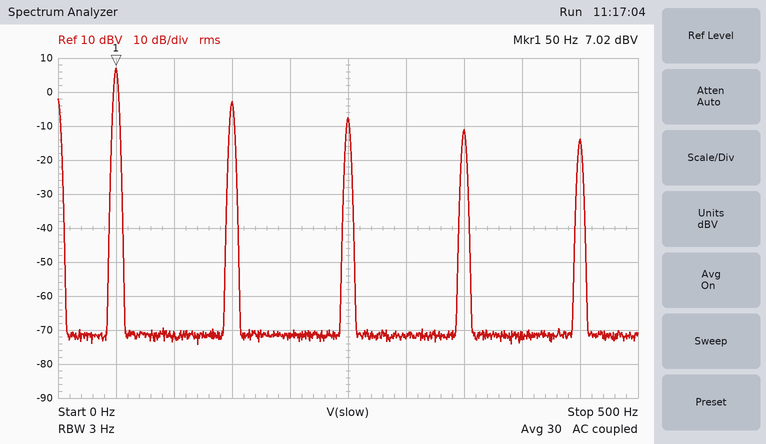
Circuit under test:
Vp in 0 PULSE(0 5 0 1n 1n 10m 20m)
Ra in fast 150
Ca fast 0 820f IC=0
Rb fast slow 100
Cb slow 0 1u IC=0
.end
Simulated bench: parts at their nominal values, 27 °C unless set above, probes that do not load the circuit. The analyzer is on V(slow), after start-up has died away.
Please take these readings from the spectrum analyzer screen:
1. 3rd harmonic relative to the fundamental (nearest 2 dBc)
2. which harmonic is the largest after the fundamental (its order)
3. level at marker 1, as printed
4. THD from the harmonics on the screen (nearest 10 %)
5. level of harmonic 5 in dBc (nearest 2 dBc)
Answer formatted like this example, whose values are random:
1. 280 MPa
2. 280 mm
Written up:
1. -10 dBc
2. 3
3. 7.02 dBV
4. 40 %
5. -14 dBc
